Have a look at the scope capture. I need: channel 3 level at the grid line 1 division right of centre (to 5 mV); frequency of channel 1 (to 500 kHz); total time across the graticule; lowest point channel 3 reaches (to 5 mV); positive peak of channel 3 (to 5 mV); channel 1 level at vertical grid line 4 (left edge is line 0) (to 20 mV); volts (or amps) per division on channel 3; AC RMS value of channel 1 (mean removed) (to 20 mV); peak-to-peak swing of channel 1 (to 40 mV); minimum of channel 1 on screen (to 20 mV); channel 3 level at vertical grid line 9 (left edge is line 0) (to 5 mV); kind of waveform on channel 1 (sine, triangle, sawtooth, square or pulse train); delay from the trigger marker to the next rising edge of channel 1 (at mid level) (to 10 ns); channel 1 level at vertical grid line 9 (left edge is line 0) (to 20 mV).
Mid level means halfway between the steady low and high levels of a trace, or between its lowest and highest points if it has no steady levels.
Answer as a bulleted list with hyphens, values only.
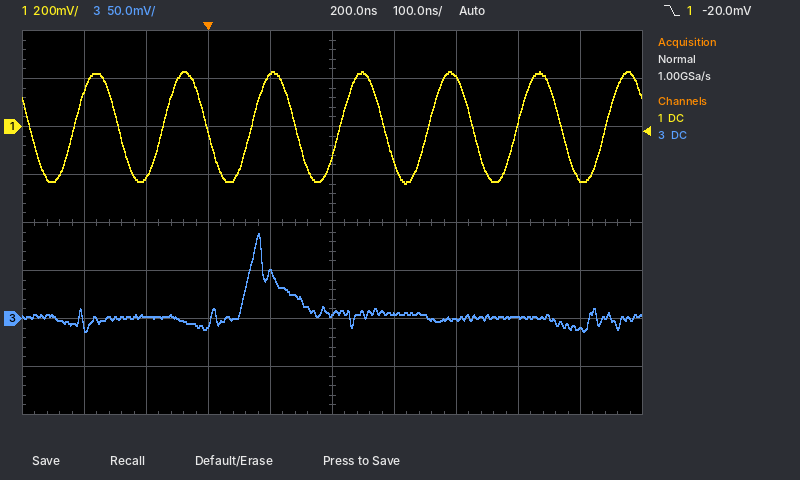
- 5 mV
- 7.0 MHz
- 1 µs
- -15 mV
- 90 mV
- 220 mV
- 50 mV
- 160 mV
- 480 mV
- -240 mV
- -10 mV
- sine
- 70 ns
- -220 mV
